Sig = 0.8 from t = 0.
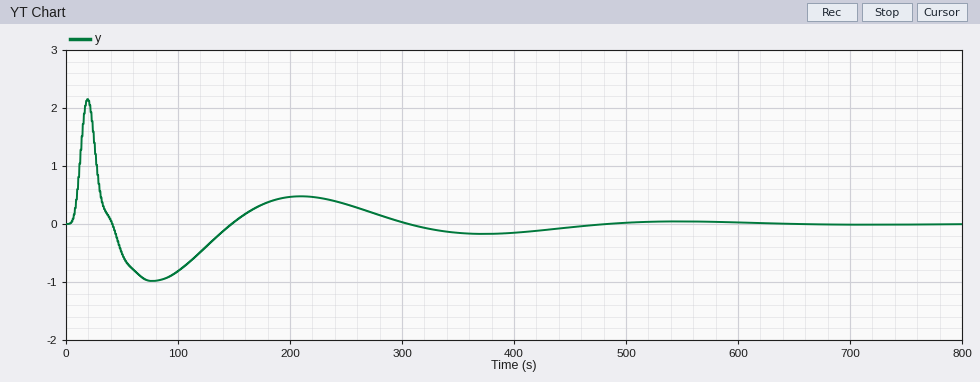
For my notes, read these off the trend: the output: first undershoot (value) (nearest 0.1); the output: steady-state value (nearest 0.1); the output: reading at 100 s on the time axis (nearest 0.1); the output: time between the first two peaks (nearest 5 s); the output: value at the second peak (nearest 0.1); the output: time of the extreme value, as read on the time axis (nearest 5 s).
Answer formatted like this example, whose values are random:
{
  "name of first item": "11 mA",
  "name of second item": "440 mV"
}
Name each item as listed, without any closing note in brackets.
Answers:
{
  "the output: first undershoot (value)": "-1.0",
  "the output: steady-state value": "0.0",
  "the output: reading at 100 s on the time axis": "-0.8",
  "the output: time between the first two peaks": "190 s",
  "the output: value at the second peak": "0.5",
  "the output: time of the extreme value, as read on the time axis": "20 s"
}
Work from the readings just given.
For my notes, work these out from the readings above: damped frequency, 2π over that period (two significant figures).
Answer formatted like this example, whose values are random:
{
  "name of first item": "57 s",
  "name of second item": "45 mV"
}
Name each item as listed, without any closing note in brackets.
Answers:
{
  "damped frequency, 2π over that period": "0.033 rad/s"
}
